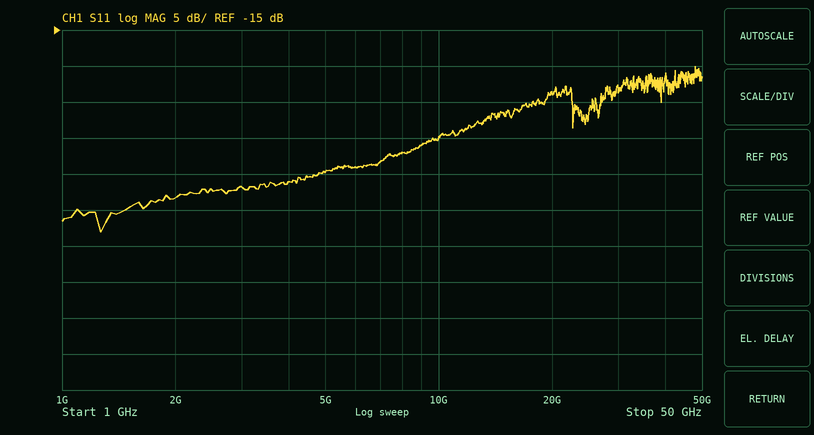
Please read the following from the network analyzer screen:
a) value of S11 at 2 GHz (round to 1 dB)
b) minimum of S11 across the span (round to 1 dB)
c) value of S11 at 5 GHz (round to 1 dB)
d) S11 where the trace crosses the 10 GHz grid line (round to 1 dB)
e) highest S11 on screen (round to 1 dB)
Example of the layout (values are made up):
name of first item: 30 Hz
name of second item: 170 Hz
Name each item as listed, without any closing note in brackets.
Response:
value of S11 at 2 GHz: -38 dB
minimum of S11 across the span: -43 dB
value of S11 at 5 GHz: -35 dB
S11 where the trace crosses the 10 GHz grid line: -30 dB
highest S11 on screen: -20 dB
